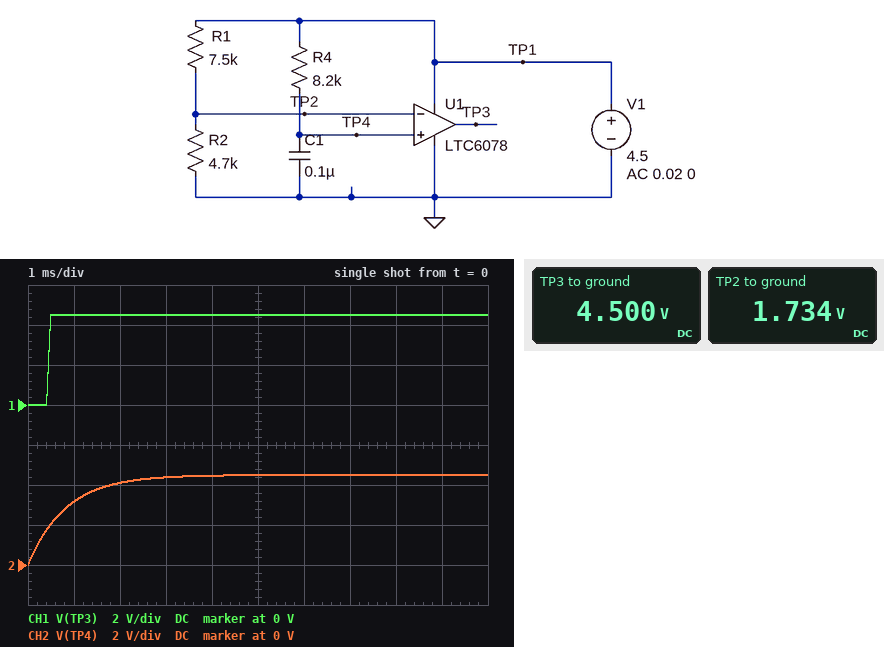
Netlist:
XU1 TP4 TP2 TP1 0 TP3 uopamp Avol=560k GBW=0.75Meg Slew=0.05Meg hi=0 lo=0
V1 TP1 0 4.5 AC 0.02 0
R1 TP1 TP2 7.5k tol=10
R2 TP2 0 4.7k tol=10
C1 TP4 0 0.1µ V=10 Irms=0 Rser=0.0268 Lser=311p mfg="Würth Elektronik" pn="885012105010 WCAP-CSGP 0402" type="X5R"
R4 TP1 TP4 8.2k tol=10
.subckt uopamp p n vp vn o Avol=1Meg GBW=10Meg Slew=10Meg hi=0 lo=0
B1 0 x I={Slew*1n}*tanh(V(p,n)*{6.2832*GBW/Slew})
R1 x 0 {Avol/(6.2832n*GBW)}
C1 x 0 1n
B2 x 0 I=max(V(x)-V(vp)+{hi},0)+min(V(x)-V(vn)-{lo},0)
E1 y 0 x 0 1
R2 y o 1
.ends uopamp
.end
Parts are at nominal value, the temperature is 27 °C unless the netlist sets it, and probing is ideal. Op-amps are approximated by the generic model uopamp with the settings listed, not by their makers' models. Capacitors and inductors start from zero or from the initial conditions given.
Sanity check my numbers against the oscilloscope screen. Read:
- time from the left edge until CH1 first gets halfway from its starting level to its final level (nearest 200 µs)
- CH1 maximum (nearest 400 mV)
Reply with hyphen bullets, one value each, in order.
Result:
- 400 µs
- 4.4 V
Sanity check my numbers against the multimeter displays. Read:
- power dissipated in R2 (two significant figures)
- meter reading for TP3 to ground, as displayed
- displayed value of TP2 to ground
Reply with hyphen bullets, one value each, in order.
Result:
- 640 µW
- 4.500 V
- 1.734 V
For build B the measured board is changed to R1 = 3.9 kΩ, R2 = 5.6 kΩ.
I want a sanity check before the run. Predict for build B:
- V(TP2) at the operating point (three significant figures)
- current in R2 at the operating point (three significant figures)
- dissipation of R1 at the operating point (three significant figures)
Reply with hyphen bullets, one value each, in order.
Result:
- 2.65 V
- 474 µA
- 875 µW
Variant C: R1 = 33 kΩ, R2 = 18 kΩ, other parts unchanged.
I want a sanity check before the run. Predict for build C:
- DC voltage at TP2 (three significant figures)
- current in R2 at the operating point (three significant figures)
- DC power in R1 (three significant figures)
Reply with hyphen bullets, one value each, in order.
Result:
- 1.59 V
- 88.2 µA
- 257 µW
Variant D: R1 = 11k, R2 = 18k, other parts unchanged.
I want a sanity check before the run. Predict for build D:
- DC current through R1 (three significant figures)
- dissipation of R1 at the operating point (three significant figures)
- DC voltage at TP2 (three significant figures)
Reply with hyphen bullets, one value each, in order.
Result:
- 155 µA
- 265 µW
- 2.79 V
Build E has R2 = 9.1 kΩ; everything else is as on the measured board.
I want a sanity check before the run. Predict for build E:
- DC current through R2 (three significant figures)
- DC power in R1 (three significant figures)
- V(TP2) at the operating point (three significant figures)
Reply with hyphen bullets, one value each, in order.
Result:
- 271 µA
- 551 µW
- 2.47 V
